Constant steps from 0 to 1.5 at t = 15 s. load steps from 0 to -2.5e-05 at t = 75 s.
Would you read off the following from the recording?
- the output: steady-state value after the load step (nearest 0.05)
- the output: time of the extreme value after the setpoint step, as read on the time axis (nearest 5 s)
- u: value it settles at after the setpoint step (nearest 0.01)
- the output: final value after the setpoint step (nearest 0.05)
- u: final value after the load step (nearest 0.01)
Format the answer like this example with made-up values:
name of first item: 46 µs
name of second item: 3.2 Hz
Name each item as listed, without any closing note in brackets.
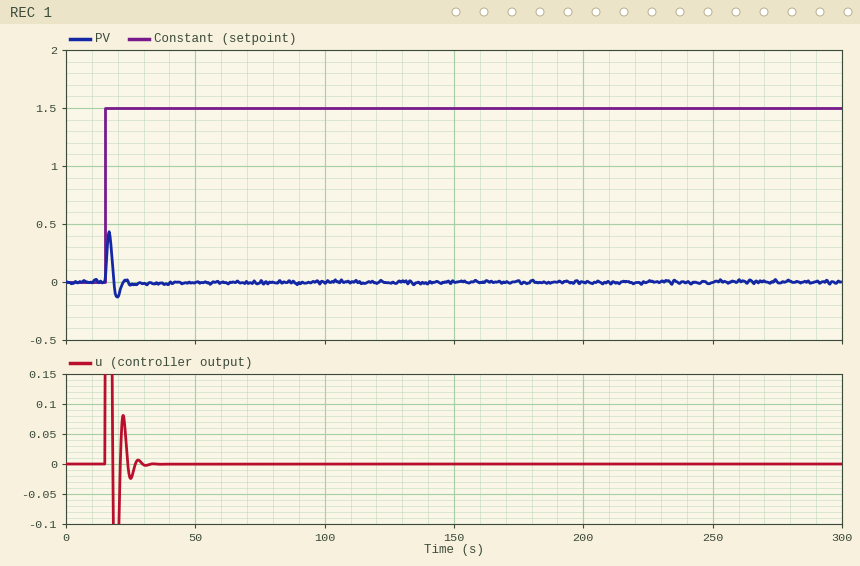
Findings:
the output: steady-state value after the load step: 0.00
the output: time of the extreme value after the setpoint step, as read on the time axis: 15 s
u: value it settles at after the setpoint step: 0.00
the output: final value after the setpoint step: 0.00
u: final value after the load step: 0.00
